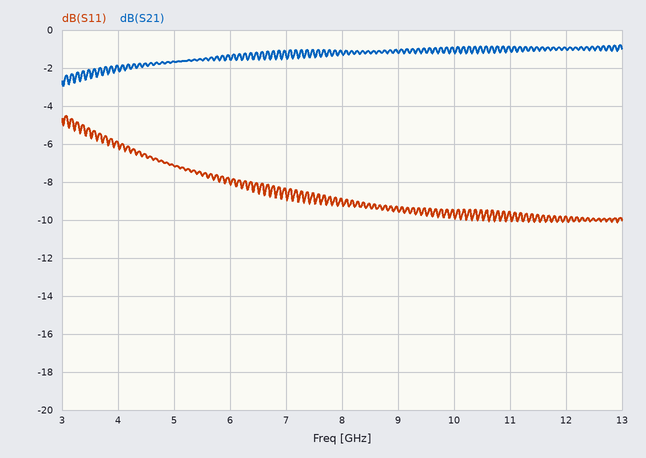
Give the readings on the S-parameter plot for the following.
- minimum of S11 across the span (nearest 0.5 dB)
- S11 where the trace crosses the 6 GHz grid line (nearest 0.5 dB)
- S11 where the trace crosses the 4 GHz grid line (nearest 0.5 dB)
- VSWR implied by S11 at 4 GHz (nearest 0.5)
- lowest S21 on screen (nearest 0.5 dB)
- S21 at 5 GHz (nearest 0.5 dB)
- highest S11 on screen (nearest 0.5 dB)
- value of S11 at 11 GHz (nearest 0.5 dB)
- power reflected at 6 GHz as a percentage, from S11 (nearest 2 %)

-10.0 dB
-8.0 dB
-6.0 dB
3.0
-3.0 dB
-1.5 dB
-4.5 dB
-9.5 dB
16 %
